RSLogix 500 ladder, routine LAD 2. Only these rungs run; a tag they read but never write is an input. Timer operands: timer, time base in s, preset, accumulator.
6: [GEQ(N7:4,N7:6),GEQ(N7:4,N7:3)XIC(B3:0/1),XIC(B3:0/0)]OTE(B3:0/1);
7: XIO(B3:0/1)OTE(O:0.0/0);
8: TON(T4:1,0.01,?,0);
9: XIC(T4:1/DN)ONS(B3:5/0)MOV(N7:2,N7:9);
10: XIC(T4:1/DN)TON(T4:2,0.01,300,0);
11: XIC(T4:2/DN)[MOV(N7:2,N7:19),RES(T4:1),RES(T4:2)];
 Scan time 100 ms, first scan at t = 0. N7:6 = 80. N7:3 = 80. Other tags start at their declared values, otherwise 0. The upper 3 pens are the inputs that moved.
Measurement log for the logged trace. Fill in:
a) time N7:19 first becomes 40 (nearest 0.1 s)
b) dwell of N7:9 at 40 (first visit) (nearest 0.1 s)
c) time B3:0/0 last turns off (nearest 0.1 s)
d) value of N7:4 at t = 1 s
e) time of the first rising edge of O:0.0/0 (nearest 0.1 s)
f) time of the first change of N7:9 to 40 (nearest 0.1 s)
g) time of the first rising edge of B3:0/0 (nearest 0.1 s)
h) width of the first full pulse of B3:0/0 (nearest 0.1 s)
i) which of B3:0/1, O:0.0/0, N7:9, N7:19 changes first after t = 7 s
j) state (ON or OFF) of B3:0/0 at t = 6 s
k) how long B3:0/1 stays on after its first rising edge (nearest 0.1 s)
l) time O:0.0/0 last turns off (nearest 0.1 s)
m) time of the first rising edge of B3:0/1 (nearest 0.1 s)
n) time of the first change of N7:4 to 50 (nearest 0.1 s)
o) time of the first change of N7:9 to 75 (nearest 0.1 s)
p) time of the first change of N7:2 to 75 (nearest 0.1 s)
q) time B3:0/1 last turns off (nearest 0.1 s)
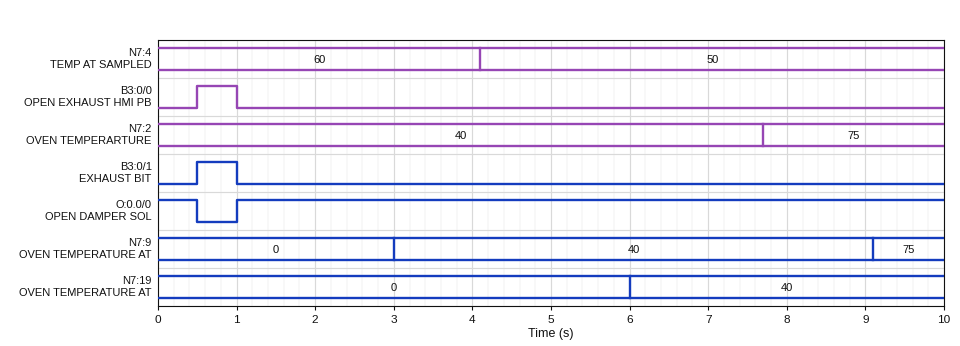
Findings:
6.0 s
6.1 s
1.0 s
60
1.0 s
3.0 s
0.5 s
0.5 s
N7:9
OFF
0.5 s
0.5 s
0.5 s
4.1 s
9.1 s
7.7 s
1.0 s
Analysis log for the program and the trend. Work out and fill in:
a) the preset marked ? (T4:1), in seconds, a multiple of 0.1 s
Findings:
3.0 s
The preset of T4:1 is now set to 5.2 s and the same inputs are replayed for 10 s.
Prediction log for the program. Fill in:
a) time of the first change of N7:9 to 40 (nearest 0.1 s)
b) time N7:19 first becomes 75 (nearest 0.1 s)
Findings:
5.2 s
8.2 s
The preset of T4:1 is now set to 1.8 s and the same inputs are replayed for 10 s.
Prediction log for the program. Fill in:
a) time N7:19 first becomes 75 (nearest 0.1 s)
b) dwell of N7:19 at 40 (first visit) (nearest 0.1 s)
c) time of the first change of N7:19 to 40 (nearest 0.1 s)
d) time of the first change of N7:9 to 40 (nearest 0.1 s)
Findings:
9.7 s
4.9 s
4.8 s
1.8 s
